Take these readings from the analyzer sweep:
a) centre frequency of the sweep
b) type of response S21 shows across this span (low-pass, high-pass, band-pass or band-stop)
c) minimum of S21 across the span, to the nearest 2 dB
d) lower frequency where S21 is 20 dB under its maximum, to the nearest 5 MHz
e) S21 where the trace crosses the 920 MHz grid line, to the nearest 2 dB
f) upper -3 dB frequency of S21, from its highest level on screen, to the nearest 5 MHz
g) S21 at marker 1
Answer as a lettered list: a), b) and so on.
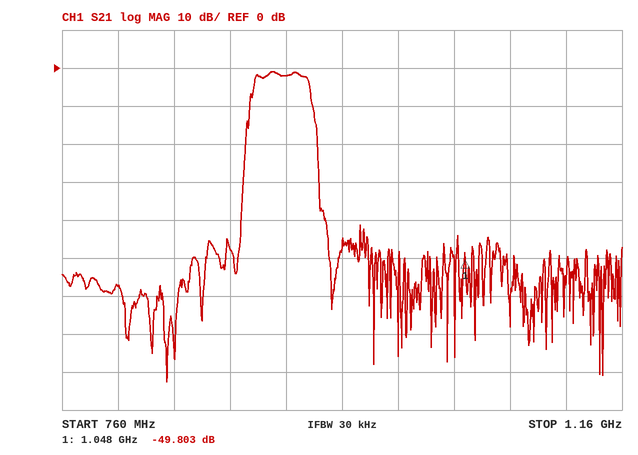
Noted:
a) 960 MHz
b) band-pass
c) -82 dB
d) 890 MHz
e) -2 dB
f) 935 MHz
g) -49.803 dB
